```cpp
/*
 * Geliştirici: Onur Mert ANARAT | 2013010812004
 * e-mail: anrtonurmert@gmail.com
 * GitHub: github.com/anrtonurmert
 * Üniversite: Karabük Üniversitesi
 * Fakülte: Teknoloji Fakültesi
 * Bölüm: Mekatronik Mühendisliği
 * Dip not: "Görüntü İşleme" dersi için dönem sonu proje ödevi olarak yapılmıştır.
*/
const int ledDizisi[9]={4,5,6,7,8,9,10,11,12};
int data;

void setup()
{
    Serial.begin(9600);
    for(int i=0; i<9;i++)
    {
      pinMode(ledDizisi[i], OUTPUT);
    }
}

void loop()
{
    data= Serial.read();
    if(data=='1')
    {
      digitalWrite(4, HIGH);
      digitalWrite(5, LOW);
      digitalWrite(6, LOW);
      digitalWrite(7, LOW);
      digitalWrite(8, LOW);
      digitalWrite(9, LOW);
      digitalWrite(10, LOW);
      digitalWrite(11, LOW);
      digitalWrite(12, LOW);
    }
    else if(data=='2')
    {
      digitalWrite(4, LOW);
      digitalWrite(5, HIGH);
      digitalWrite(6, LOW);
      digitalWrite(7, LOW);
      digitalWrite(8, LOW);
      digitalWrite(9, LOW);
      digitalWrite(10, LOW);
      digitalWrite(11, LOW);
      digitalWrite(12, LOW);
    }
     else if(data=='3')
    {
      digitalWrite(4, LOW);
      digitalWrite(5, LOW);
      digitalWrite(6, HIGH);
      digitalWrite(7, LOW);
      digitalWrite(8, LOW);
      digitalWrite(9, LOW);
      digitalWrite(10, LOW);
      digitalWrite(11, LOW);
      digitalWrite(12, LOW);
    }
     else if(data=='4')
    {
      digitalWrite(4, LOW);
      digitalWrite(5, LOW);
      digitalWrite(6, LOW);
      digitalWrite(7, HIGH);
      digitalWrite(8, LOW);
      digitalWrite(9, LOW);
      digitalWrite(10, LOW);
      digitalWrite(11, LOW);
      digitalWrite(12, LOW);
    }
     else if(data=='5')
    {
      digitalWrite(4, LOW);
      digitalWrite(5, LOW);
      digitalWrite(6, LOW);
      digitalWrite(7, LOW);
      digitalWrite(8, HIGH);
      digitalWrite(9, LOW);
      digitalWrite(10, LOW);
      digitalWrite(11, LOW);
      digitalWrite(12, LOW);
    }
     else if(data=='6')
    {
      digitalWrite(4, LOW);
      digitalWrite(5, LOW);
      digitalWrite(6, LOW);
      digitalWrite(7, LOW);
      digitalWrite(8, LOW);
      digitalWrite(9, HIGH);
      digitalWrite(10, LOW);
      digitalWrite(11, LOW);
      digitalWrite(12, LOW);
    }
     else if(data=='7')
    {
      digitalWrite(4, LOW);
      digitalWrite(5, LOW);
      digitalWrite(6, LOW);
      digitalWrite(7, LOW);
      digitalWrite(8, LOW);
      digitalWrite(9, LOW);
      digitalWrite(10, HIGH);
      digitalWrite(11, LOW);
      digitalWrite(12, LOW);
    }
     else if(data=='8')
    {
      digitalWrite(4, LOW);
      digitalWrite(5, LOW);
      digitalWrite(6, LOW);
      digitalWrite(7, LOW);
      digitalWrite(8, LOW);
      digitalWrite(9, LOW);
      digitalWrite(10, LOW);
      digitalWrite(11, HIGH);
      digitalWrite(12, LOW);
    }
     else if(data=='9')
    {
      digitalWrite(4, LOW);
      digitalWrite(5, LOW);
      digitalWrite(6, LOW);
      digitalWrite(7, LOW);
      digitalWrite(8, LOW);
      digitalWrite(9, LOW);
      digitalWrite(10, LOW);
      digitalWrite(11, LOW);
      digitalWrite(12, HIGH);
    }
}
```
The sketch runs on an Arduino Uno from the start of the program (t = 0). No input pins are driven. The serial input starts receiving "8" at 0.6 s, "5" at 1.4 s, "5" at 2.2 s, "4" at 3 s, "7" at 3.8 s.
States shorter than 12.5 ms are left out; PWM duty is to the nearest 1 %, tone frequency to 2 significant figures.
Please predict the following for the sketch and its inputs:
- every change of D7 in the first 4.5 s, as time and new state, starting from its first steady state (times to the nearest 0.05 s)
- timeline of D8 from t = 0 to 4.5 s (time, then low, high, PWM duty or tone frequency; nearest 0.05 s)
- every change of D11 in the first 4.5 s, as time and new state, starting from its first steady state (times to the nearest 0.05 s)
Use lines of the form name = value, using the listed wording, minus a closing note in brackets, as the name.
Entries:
every change of D7 in the first 4.5 s, as time and new state, starting from its first steady state = 0 s low; 3 s high; 3.8 s low
timeline of D8 from t = 0 to 4.5 s = 0 s low; 1.4 s high; 3 s low
every change of D11 in the first 4.5 s, as time and new state, starting from its first steady state = 0 s low; 0.6 s high; 1.4 s low
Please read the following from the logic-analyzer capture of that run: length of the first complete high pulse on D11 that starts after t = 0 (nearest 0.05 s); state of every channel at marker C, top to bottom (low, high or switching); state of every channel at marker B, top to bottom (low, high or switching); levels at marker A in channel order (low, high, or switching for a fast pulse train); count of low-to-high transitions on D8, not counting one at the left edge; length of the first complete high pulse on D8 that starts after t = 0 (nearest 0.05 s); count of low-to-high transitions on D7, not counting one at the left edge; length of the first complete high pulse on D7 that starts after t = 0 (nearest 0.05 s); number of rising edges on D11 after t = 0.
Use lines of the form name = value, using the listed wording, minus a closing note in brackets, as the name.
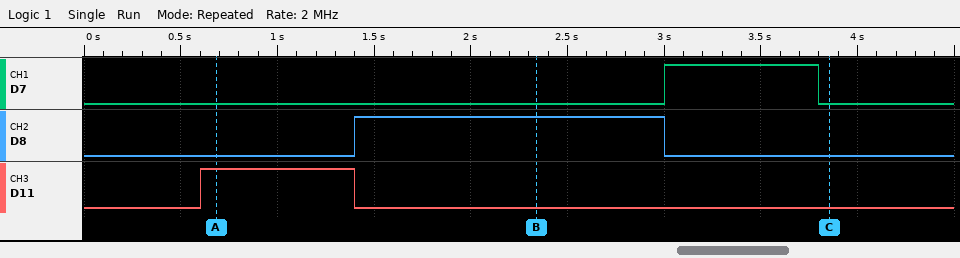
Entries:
length of the first complete high pulse on D11 that starts after t = 0 = 0.80 s
state of every channel at marker C, top to bottom = D7 low, D8 low, D11 low
state of every channel at marker B, top to bottom = D7 low, D8 high, D11 low
levels at marker A in channel order = D7 low, D8 low, D11 high
count of low-to-high transitions on D8, not counting one at the left edge = 1
length of the first complete high pulse on D8 that starts after t = 0 = 1.60 s
count of low-to-high transitions on D7, not counting one at the left edge = 1
length of the first complete high pulse on D7 that starts after t = 0 = 0.80 s
number of rising edges on D11 after t = 0 = 1
